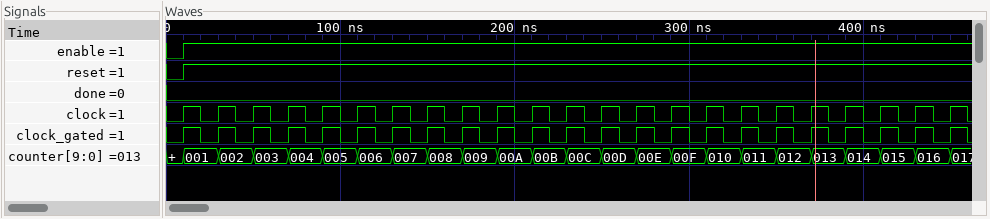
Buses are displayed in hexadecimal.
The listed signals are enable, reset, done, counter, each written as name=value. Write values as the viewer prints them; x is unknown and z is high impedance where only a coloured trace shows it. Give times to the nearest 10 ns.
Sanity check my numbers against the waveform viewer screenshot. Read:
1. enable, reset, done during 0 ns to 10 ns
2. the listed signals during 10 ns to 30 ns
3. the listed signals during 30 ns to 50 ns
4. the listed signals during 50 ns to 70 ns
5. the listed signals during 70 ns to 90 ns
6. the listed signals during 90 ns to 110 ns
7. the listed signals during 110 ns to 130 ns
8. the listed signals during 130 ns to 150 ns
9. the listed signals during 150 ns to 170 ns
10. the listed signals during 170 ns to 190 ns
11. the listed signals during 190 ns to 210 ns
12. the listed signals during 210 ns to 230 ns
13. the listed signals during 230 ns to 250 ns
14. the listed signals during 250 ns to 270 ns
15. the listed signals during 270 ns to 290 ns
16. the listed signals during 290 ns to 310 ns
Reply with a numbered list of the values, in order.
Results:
1. enable=0, reset=0, done=0
2. enable=1, reset=1, done=0, counter=001
3. enable=1, reset=1, done=0, counter=002
4. enable=1, reset=1, done=0, counter=003
5. enable=1, reset=1, done=0, counter=004
6. enable=1, reset=1, done=0, counter=005
7. enable=1, reset=1, done=0, counter=006
8. enable=1, reset=1, done=0, counter=007
9. enable=1, reset=1, done=0, counter=008
10. enable=1, reset=1, done=0, counter=009
11. enable=1, reset=1, done=0, counter=00A
12. enable=1, reset=1, done=0, counter=00B
13. enable=1, reset=1, done=0, counter=00C
14. enable=1, reset=1, done=0, counter=00D
15. enable=1, reset=1, done=0, counter=00E
16. enable=1, reset=1, done=0, counter=00F
